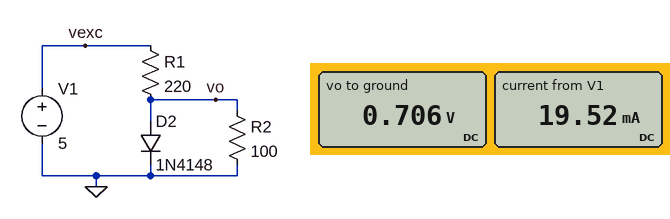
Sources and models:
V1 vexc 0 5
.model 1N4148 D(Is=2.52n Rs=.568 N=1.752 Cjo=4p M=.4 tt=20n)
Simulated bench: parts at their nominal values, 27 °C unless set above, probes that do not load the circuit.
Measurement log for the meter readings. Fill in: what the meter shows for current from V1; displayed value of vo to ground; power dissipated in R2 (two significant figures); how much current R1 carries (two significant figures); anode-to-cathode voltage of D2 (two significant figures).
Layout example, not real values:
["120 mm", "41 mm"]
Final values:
["19.52 mA", "0.706 V", "5.0 mW", "20 mA", "710 mV"]
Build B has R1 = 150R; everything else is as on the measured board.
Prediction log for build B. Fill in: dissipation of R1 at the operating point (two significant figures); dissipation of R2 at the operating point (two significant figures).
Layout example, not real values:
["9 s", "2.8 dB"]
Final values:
["120 mW", "5.4 mW"]
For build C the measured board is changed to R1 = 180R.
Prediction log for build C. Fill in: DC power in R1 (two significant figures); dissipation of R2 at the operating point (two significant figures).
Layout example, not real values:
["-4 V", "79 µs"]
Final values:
["100 mW", "5.2 mW"]
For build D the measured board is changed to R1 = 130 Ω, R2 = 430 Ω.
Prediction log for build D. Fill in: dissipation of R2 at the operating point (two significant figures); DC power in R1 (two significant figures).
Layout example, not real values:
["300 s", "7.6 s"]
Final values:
["1.3 mW", "140 mW"]
